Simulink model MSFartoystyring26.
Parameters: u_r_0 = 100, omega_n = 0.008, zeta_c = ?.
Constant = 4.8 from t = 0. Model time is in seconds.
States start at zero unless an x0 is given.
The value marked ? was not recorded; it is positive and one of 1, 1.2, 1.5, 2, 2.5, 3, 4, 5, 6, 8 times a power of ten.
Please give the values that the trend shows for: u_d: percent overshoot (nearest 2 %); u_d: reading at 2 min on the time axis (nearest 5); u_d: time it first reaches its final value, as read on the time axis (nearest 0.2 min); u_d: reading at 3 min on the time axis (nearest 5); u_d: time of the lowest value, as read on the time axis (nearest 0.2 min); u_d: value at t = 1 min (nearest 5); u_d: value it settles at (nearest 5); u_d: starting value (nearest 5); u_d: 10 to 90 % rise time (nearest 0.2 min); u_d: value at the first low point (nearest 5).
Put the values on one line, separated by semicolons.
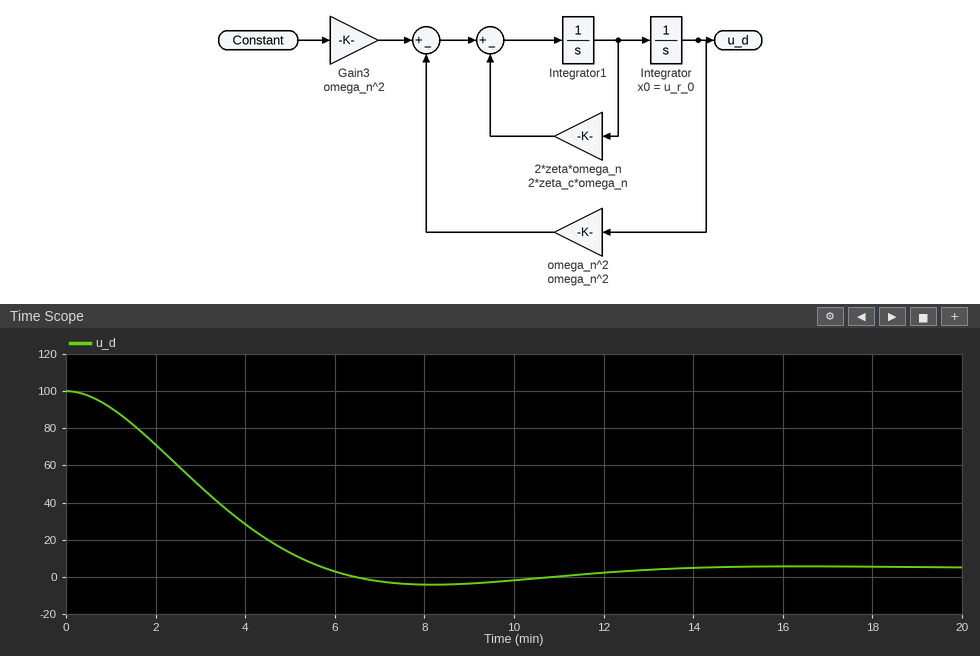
10 %; 70; 5.8 min; 50; 8.2 min; 90; 5; 100; 3.8 min; -5
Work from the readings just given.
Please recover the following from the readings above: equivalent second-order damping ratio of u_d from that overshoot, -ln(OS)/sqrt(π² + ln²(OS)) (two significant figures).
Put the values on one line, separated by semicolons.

0.59
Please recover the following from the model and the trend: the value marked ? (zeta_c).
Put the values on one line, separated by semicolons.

0.6
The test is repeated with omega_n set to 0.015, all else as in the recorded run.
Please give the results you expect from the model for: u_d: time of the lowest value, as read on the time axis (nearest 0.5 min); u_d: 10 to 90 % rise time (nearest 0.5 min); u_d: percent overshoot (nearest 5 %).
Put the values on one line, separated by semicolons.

4.5 min; 2.0 min; 10 %
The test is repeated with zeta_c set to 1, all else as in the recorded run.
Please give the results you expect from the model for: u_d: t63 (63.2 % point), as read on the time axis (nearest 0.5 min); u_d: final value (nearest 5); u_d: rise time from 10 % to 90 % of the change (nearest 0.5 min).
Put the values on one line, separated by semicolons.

4.5 min; 5; 7.0 min
